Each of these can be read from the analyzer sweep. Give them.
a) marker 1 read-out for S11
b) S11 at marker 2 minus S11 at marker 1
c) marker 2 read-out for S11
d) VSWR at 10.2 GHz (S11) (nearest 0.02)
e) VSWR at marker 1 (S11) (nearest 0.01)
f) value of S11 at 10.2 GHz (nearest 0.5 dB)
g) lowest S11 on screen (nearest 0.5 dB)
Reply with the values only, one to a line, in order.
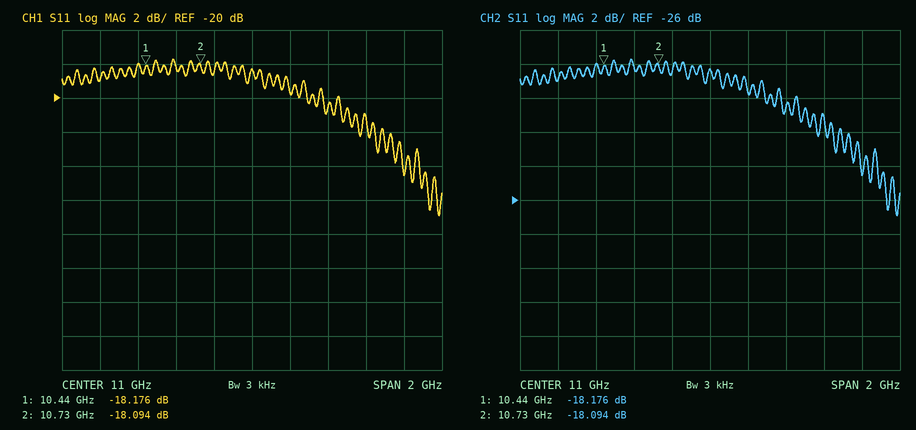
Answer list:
-18.176 dB
0.082 dB
-18.094 dB
1.26
1.28
-19.0 dB
-27.0 dB
